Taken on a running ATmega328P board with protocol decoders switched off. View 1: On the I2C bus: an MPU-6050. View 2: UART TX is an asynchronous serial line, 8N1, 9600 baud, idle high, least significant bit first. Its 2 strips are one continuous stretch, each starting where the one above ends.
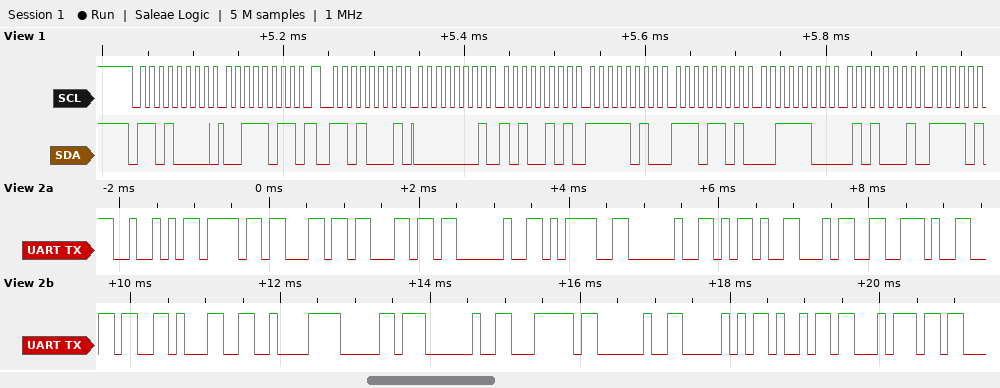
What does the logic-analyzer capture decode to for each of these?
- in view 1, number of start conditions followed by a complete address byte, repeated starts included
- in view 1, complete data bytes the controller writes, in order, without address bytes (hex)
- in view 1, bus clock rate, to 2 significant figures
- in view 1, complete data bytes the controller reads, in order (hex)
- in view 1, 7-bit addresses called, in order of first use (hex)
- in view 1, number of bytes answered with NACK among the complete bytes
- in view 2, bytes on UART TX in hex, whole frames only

2
3B
100 kHz
01 A5 FA ED 3C 51
0x68
0
52 6F 6C 6C 20 3D 20 2D 34 2E 36 31 C2 B0 20 7C 20 50 69 74
